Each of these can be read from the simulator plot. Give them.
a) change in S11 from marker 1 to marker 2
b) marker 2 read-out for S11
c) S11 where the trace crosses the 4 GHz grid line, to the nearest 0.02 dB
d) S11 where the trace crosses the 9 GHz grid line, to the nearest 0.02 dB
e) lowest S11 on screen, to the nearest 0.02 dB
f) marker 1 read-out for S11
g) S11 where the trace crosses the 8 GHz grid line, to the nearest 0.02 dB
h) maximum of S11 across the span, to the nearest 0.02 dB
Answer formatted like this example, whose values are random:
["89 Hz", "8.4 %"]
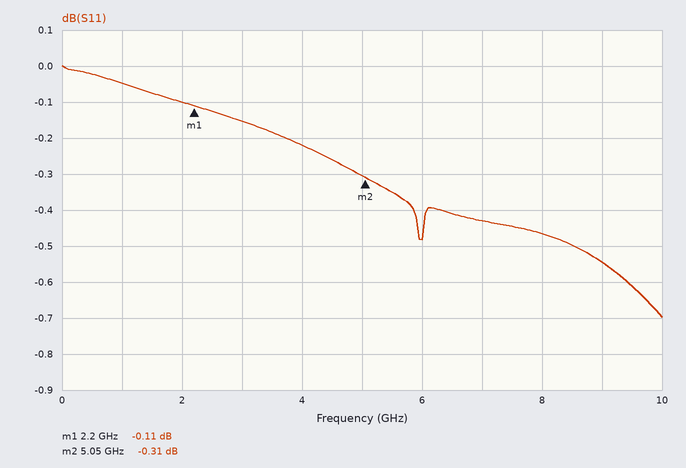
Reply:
["-0.20 dB", "-0.31 dB", "-0.22 dB", "-0.54 dB", "-0.70 dB", "-0.11 dB", "-0.46 dB", "0.00 dB"]
